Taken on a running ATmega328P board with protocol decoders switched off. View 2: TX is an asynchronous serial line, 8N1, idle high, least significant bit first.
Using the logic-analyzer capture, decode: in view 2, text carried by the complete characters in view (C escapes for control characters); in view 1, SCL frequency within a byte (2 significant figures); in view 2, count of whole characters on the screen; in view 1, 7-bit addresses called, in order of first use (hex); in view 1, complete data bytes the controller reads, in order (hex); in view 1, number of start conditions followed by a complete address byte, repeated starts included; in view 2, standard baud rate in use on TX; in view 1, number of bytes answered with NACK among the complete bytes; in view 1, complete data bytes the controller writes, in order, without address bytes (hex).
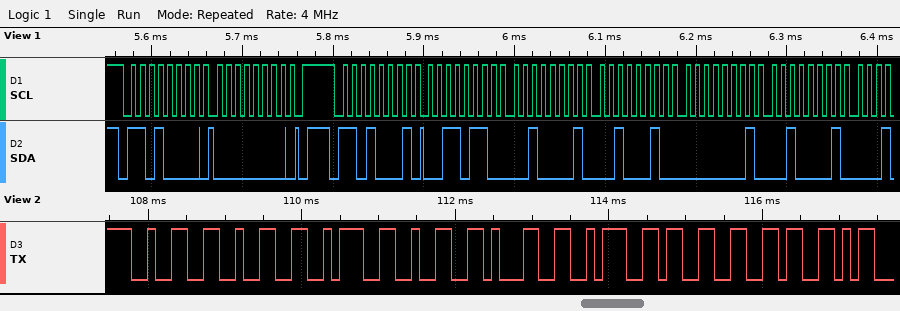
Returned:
"22:21:36"
100 kHz
8
0x68
36 21 22 01 21
2
9600 baud
0
00
